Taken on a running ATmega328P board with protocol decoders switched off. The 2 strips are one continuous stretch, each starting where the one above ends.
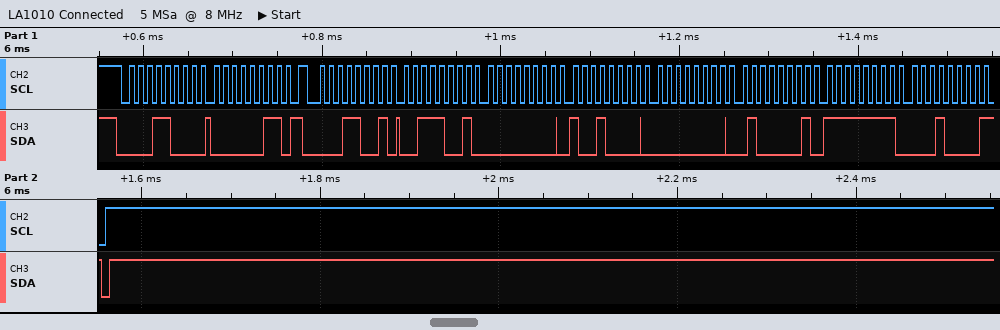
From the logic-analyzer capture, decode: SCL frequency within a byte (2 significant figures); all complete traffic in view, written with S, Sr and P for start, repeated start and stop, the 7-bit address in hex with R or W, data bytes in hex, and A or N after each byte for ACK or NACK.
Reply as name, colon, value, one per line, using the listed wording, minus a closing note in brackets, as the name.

SCL frequency within a byte: 100 kHz
all complete traffic in view, written with S, Sr and P for start, repeated start and stop, the 7-bit address in hex with R or W, data bytes in hex, and A or N after each byte for ACK or NACK: S 0CW A 03 A Sr 0CR A 39 A 00 A 90 A 00 A 41 A FF A 10 N P
